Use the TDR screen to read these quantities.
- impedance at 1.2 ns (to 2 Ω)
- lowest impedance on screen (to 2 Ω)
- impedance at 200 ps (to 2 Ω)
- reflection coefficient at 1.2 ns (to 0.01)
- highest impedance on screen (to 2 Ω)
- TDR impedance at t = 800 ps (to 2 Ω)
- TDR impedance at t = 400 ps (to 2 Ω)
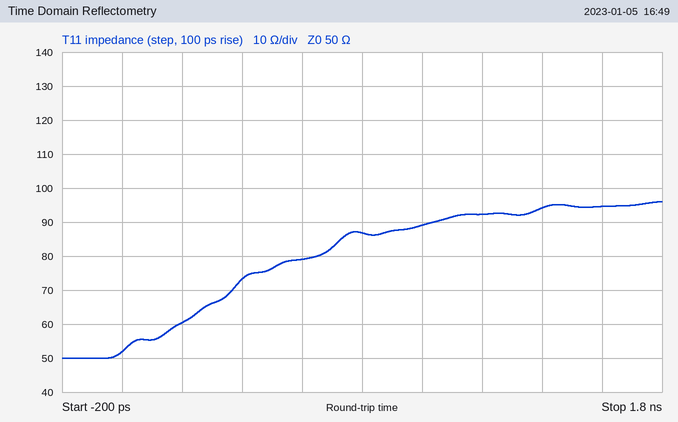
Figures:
92 Ω
50 Ω
60 Ω
+0.30
96 Ω
86 Ω
74 Ω
